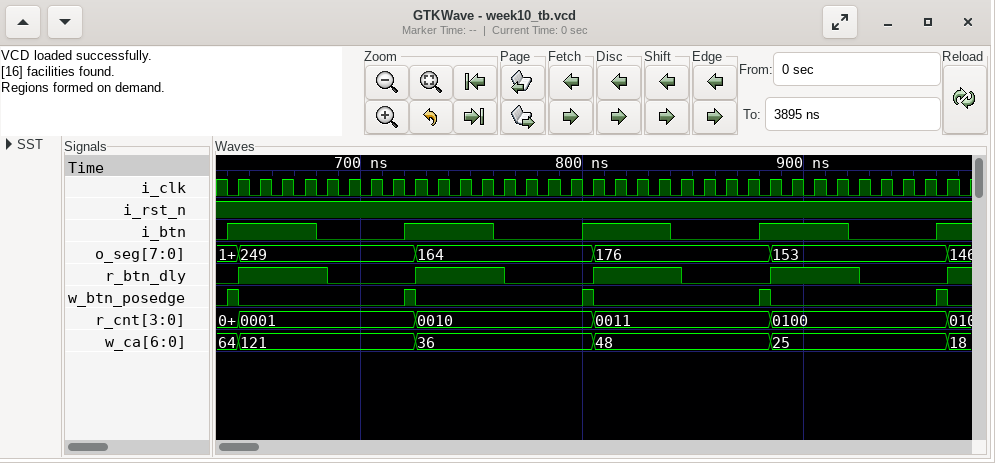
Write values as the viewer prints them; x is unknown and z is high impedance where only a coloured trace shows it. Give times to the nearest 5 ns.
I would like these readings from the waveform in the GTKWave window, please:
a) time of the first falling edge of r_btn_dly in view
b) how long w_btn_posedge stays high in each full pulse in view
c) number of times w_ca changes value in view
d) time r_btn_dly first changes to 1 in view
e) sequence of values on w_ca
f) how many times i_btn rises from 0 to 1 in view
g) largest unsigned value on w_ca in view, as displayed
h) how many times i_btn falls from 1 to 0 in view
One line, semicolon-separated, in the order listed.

685 ns; 5 ns, 5 ns, 5 ns, 5 ns, 5 ns; 5; 645 ns; 64, 121, 36, 48, 25, 18; 5; 121; 4
